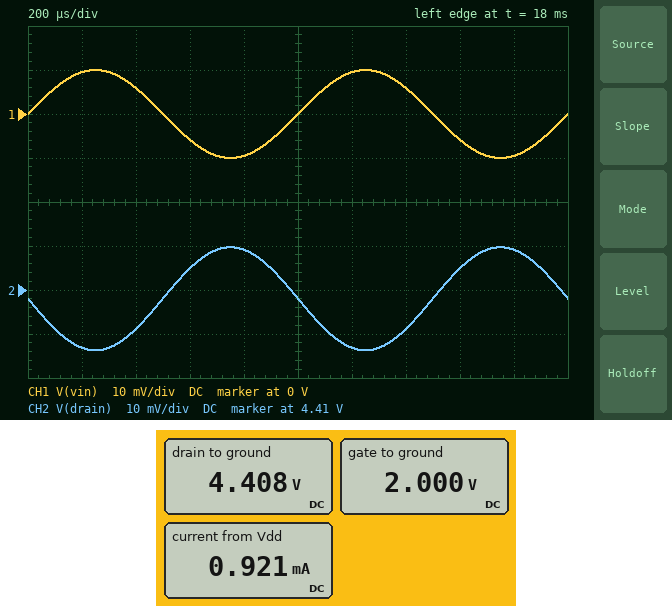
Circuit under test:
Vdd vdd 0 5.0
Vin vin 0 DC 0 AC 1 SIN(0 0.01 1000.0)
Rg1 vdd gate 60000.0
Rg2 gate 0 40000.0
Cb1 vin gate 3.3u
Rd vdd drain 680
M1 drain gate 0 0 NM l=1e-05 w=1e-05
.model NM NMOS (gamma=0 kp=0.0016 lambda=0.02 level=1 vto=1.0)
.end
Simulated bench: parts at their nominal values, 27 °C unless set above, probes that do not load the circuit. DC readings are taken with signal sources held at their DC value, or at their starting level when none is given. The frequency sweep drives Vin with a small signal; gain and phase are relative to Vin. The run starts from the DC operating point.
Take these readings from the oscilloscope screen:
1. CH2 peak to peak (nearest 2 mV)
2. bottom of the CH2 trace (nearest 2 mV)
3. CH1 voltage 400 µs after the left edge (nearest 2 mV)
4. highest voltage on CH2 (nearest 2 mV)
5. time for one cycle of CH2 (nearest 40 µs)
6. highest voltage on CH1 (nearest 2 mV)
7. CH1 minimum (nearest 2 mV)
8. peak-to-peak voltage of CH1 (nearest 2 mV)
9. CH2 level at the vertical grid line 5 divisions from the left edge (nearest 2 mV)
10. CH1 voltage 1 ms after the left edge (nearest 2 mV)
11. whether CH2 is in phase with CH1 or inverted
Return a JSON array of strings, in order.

["24 mV", "4.396 V", "6 mV", "4.420 V", "1.00 ms", "10 mV", "-10 mV", "20 mV", "4.408 V", "0 V", "inverted"]
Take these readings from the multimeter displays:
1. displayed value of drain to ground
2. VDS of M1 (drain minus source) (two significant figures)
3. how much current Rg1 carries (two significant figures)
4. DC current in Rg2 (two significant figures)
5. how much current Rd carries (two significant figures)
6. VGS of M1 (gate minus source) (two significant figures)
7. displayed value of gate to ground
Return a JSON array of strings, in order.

["4.408 V", "4.4 V", "50 µA", "50 µA", "870 µA", "2.0 V", "2.000 V"]
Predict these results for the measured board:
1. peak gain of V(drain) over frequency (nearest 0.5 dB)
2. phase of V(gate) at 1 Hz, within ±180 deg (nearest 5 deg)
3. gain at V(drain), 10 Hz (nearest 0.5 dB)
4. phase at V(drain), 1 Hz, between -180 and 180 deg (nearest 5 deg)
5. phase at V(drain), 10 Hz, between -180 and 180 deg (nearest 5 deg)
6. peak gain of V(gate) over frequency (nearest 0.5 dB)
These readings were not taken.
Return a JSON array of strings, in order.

["1.5 dB", "65 deg", "1.0 dB", "-115 deg", "-170 deg", "0 dB"]
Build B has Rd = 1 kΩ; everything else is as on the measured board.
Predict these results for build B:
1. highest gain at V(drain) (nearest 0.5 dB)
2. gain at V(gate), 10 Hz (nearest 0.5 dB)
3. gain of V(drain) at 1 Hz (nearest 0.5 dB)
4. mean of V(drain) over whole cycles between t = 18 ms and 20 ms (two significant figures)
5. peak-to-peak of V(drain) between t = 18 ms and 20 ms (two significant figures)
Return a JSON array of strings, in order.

["4.5 dB", "0 dB", "-2.5 dB", "4.1 V", "34 mV"]
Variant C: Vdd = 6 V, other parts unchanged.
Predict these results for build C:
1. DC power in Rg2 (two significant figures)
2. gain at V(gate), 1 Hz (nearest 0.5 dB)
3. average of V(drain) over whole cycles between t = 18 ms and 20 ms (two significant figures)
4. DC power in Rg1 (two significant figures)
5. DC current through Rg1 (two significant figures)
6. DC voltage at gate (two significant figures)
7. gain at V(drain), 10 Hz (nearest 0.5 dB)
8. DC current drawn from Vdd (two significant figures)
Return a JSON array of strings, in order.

["140 µW", "-7.0 dB", "4.8 V", "220 µW", "60 µA", "2.4 V", "4.0 dB", "1.8 mA"]
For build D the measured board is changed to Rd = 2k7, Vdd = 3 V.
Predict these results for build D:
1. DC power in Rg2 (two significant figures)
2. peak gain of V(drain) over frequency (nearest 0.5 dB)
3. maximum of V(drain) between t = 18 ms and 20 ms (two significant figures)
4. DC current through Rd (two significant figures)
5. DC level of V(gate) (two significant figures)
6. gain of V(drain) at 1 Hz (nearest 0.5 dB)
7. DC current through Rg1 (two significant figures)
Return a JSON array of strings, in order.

["36 µW", "-1.0 dB", "2.9 V", "34 µA", "1.2 V", "-8.0 dB", "30 µA"]
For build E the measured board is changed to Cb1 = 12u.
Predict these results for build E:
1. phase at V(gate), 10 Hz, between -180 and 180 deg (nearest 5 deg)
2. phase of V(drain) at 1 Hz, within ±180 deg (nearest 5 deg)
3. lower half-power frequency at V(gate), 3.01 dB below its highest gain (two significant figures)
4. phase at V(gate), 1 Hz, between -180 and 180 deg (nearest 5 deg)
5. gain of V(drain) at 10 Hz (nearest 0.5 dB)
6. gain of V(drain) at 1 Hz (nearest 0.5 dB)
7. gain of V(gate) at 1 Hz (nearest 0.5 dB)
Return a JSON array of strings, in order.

["5 deg", "-150 deg", "550 mHz", "30 deg", "1.5 dB", "0 dB", "-1.0 dB"]
